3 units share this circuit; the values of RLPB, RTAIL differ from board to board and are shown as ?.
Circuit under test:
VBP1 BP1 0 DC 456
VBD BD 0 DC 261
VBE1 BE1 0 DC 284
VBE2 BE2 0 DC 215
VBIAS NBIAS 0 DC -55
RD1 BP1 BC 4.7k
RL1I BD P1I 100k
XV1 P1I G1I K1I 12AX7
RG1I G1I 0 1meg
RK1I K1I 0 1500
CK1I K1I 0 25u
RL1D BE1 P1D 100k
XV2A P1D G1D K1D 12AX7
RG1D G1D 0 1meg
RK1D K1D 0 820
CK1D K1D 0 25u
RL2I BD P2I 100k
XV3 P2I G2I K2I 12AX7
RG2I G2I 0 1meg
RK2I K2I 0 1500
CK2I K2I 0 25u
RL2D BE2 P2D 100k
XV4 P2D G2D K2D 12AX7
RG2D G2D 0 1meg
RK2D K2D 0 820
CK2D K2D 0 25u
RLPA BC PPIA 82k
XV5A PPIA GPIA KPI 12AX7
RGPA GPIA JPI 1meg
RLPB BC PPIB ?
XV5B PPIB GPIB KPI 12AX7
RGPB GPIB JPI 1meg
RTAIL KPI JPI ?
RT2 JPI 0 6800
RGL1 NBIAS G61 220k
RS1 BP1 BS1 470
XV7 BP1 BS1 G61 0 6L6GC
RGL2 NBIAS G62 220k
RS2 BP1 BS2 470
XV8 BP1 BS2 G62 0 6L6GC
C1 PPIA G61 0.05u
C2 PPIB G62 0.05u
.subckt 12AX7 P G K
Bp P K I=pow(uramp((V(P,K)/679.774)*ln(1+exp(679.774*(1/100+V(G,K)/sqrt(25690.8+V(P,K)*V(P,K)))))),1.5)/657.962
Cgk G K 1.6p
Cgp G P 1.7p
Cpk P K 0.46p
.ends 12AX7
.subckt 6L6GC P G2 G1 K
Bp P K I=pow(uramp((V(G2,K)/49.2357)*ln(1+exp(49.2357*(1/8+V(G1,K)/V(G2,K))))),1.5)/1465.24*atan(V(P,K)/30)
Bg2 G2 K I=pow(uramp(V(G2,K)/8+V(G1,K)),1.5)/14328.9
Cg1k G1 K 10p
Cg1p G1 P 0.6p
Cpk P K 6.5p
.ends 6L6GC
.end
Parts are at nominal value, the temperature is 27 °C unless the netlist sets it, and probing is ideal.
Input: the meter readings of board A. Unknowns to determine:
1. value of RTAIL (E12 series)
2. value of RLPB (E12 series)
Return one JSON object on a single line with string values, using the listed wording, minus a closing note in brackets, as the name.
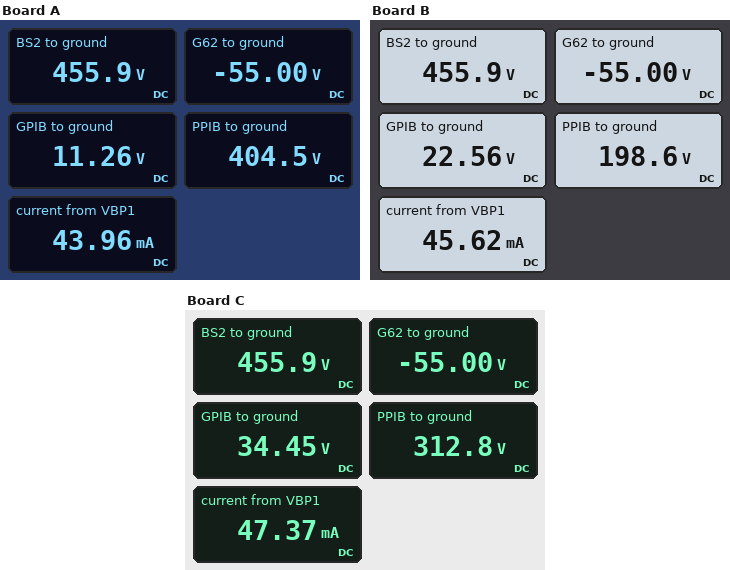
{"value of RTAIL": "2.2 kΩ", "value of RLPB": "47 kΩ"}
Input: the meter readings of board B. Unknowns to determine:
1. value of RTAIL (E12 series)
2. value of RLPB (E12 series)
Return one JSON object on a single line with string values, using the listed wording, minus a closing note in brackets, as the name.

{"value of RTAIL": "390 Ω", "value of RLPB": "220 kΩ"}
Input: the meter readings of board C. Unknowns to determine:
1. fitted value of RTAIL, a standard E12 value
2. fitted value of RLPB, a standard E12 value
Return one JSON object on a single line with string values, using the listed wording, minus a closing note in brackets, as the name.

{"fitted value of RTAIL, a standard E12 value": "270 Ω", "fitted value of RLPB, a standard E12 value": "39 kΩ"}
